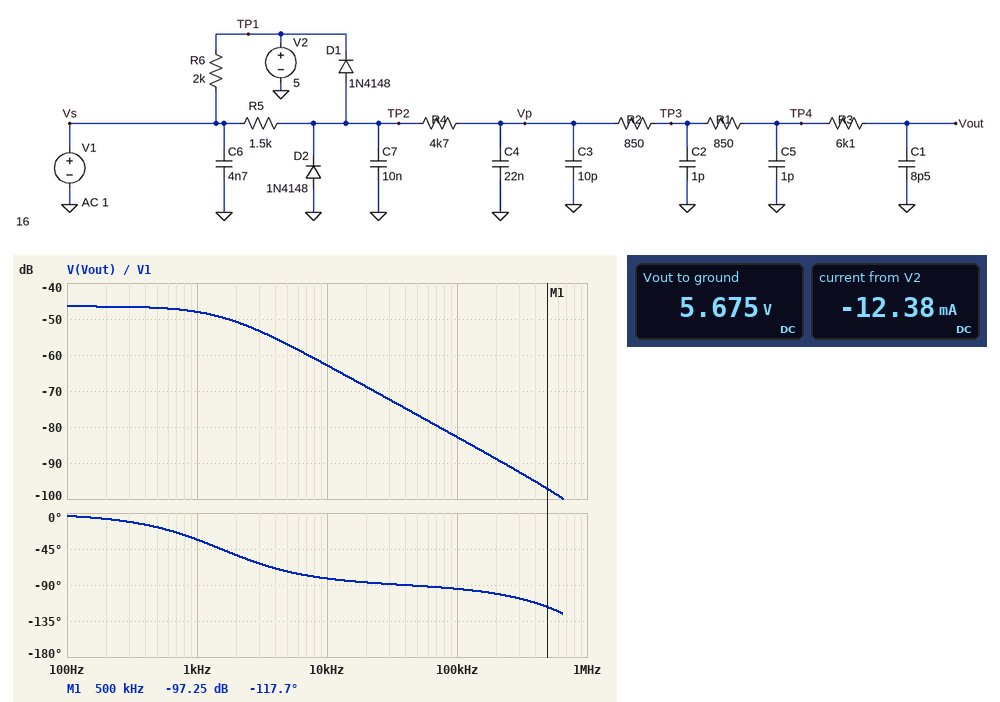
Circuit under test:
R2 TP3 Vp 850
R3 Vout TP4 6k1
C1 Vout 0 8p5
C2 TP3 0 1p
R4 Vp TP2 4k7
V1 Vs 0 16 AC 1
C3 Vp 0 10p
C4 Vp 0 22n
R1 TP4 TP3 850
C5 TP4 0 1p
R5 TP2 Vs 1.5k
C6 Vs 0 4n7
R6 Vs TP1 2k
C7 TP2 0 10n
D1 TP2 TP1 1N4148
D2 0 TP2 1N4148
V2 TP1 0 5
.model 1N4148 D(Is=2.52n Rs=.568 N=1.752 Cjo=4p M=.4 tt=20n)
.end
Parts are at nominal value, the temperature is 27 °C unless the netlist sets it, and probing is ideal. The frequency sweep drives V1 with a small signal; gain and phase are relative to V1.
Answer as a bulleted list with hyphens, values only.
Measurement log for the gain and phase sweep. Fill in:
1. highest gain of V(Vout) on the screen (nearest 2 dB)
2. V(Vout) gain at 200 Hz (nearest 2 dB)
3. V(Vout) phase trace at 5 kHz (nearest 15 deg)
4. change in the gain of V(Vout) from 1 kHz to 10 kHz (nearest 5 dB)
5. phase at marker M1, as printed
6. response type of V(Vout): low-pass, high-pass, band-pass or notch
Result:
- -46 dB
- -46 dB
- -75 deg
- -15 dB
- -117.7 deg
- low-pass
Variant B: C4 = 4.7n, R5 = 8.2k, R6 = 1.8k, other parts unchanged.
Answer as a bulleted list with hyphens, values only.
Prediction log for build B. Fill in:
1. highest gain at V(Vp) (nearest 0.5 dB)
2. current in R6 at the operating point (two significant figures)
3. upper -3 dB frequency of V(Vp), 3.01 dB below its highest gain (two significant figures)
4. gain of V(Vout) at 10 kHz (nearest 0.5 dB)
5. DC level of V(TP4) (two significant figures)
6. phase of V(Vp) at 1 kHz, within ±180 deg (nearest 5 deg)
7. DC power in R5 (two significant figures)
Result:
- -47.0 dB
- 6.1 mA
- 7.1 kHz
- -52.0 dB
- 5.6 V
- -10 deg
- 13 mW
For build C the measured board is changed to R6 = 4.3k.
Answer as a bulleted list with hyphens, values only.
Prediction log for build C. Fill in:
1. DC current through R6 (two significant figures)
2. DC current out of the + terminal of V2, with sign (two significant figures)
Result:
- 2.6 mA
- -9.4 mA
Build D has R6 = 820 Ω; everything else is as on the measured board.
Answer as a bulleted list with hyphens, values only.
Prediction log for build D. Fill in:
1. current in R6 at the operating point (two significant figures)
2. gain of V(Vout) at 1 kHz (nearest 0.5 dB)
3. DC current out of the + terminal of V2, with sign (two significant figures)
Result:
- 13 mA
- -48.0 dB
- -20 mA
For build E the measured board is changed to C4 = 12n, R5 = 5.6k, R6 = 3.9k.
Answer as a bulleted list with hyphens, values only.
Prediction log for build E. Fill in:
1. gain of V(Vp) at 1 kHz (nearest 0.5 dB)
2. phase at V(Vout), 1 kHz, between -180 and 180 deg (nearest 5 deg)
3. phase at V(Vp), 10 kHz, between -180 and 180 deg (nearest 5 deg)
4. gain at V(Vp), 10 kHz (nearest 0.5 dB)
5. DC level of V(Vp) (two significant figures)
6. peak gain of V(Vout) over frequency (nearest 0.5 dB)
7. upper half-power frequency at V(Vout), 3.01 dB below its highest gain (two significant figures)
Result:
- -47.5 dB
- -20 deg
- -75 deg
- -58.5 dB
- 5.6 V
- -47.0 dB
- 2.8 kHz
